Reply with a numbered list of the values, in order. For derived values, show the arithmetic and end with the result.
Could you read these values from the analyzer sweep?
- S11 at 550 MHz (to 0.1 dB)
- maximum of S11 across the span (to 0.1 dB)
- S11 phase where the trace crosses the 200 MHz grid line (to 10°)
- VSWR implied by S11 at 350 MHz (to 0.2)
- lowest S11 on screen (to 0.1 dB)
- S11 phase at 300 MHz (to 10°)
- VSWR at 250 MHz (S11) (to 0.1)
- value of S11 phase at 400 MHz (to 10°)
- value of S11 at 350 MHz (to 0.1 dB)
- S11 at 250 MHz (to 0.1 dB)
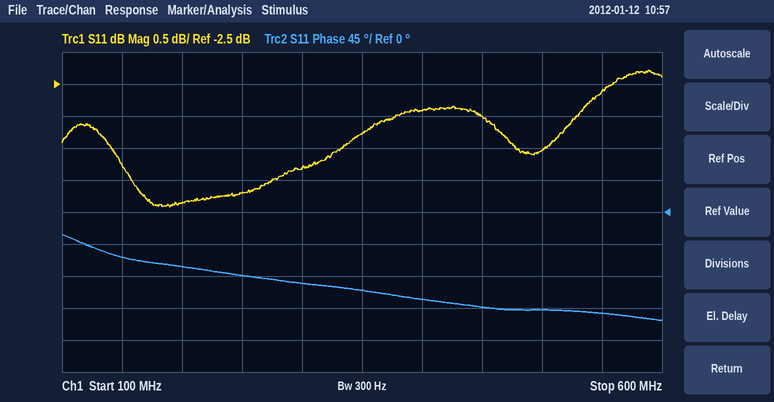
1. -2.6 dB
2. -2.3 dB
3. -80°
4. |Γ| = 10^(-3.3/20) = 0.6839; VSWR = (1 + 0.6839)/(1 − 0.6839) ≈ 5.33, so 5.4 to the nearest 0.2
5. -4.4 dB
6. -100°
7. |Γ| = 10^(-4.2/20) = 0.6166; VSWR = (1 + 0.6166)/(1 − 0.6166) ≈ 4.2
8. -120°
9. -3.3 dB
10. -4.2 dB
